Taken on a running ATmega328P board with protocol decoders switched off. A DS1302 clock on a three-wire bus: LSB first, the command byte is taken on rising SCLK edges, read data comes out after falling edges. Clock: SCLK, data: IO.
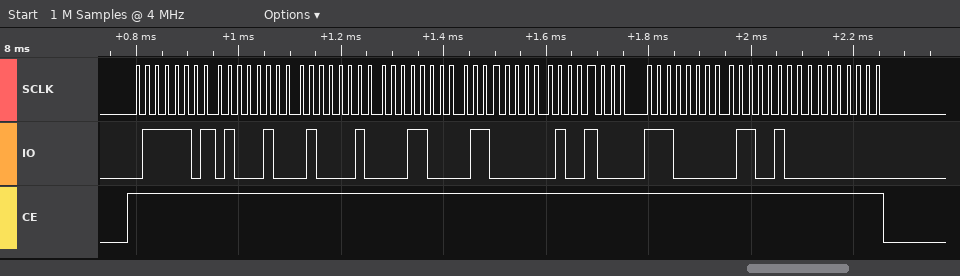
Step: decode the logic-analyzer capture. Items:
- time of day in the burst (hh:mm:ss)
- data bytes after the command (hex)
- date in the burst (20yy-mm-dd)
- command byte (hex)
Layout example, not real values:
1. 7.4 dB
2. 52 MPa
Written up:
1. 18:42:22
2. 22 42 18 06 12 07 26 00
3. 2026-12-06
4. 0xBE
